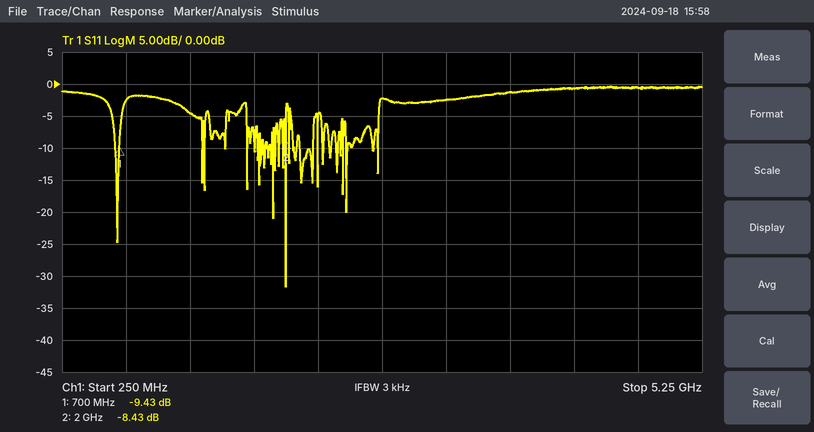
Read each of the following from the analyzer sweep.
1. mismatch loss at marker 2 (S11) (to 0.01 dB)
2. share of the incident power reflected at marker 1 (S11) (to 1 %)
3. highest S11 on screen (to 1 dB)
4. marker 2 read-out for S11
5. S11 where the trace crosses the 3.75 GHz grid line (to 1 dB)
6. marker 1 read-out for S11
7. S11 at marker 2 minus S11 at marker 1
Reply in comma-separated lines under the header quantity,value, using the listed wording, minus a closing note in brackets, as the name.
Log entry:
quantity,value
mismatch loss at marker 2 (S11),0.67 dB
share of the incident power reflected at marker 1 (S11),11 %
highest S11 on screen,0 dB
marker 2 read-out for S11,-8.43 dB
S11 where the trace crosses the 3.75 GHz grid line,-1 dB
marker 1 read-out for S11,-9.43 dB
S11 at marker 2 minus S11 at marker 1,1.00 dB
